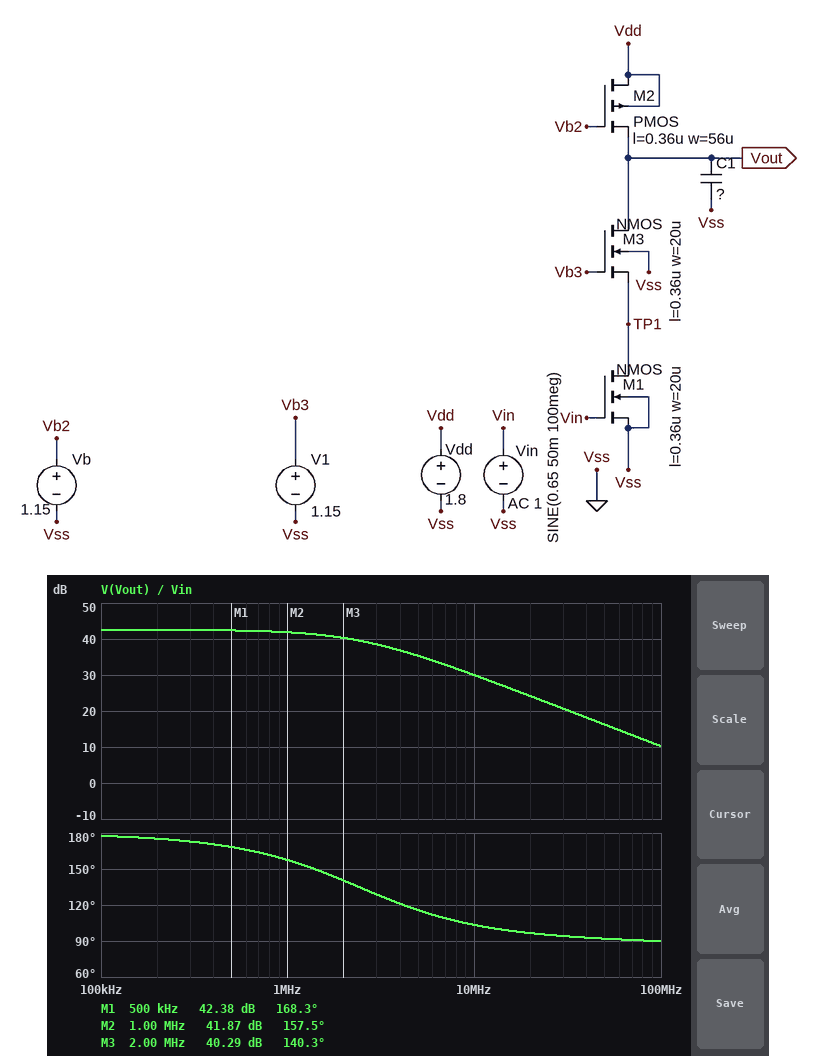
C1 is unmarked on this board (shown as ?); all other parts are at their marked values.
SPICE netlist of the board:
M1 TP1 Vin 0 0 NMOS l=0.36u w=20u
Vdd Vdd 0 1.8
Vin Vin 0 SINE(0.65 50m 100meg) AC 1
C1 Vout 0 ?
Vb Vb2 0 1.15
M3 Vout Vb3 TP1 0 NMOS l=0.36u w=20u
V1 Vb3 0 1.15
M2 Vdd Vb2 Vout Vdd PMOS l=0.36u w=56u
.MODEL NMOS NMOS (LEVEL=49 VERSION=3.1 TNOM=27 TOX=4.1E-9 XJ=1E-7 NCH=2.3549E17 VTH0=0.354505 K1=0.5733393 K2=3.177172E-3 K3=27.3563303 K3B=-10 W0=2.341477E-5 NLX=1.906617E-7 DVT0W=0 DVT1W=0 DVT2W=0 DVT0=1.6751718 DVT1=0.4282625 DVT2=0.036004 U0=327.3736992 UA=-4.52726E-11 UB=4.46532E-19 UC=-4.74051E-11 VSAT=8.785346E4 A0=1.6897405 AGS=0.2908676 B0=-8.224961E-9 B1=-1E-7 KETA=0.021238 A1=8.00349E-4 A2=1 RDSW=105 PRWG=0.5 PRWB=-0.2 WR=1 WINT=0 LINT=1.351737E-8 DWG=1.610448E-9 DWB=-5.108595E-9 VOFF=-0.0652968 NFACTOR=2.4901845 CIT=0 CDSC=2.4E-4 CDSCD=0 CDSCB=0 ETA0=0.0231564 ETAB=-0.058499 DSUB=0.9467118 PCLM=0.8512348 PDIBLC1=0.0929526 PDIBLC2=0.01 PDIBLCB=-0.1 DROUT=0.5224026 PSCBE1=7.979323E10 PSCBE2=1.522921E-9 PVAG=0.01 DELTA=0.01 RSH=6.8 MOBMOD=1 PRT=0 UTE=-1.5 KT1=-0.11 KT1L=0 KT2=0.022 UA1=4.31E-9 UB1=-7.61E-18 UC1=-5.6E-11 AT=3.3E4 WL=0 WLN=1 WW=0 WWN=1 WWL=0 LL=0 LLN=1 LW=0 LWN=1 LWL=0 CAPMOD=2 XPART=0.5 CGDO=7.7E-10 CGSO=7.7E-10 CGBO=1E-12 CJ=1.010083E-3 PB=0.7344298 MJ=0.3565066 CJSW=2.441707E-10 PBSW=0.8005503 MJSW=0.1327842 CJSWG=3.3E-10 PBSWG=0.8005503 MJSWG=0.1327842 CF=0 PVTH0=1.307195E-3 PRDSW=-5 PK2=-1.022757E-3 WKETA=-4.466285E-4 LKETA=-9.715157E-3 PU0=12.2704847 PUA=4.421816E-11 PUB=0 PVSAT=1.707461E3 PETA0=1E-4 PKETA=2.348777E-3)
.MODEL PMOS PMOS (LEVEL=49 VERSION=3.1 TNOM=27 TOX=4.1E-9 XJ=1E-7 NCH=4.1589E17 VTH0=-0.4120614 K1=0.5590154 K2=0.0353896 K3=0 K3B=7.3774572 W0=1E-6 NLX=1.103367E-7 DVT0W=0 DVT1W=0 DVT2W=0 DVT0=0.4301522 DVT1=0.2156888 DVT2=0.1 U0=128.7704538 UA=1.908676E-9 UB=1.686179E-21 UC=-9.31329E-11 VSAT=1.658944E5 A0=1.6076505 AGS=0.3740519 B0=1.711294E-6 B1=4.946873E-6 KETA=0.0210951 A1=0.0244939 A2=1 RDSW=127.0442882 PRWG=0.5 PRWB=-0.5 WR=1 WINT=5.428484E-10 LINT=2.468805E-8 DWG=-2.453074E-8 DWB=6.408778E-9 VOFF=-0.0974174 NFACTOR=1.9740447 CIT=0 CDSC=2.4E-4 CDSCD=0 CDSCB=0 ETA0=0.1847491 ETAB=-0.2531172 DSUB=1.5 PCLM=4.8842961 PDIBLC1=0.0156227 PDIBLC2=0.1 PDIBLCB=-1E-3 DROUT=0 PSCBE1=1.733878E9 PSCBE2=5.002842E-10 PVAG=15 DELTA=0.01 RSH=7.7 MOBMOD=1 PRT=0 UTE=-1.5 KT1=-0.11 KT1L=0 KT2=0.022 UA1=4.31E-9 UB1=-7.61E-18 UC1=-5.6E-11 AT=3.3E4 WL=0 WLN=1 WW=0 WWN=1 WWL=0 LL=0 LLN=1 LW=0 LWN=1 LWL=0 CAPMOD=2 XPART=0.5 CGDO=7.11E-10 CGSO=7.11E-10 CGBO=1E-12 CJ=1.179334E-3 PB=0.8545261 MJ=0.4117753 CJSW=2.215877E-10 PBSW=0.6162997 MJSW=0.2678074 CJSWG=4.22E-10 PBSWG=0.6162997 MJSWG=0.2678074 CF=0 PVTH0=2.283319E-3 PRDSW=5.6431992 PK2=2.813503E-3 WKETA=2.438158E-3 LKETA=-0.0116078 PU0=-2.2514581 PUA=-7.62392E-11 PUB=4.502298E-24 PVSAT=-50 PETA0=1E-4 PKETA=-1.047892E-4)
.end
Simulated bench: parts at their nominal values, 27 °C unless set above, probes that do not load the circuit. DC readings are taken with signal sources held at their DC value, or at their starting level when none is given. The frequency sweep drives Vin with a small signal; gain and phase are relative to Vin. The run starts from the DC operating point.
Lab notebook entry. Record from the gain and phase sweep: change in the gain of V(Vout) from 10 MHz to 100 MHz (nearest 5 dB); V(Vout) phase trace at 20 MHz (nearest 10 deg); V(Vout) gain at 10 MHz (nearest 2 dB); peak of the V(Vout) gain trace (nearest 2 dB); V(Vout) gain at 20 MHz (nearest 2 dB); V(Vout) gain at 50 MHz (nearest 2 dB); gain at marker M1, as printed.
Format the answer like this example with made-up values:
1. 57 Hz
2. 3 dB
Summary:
1. -20 dB
2. 100 deg
3. 30 dB
4. 42 dB
5. 24 dB
6. 16 dB
7. 42.38 dB
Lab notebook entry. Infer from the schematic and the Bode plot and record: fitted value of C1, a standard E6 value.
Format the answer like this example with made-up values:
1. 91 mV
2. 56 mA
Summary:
1. 1 pF
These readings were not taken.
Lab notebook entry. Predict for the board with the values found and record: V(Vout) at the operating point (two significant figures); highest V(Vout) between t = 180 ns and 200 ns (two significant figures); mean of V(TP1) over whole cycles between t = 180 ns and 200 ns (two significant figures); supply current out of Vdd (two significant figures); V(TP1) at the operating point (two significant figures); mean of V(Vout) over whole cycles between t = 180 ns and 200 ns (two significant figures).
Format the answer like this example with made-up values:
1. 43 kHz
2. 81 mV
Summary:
1. 1.0 V
2. 700 mV
3. 380 mV
4. 180 µA
5. 400 mV
6. 540 mV
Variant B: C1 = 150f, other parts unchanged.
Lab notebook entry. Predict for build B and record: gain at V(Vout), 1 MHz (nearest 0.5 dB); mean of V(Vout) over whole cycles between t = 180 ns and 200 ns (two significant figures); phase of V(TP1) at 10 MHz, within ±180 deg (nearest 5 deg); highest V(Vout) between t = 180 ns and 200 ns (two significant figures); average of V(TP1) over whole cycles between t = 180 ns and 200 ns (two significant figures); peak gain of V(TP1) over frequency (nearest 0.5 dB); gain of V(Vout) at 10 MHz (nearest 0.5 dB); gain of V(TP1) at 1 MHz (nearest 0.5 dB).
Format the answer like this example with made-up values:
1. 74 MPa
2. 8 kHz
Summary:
1. 42.5 dB
2. 780 mV
3. 160 deg
4. 1.5 V
5. 340 mV
6. 5.5 dB
7. 40.0 dB
8. 5.5 dB
